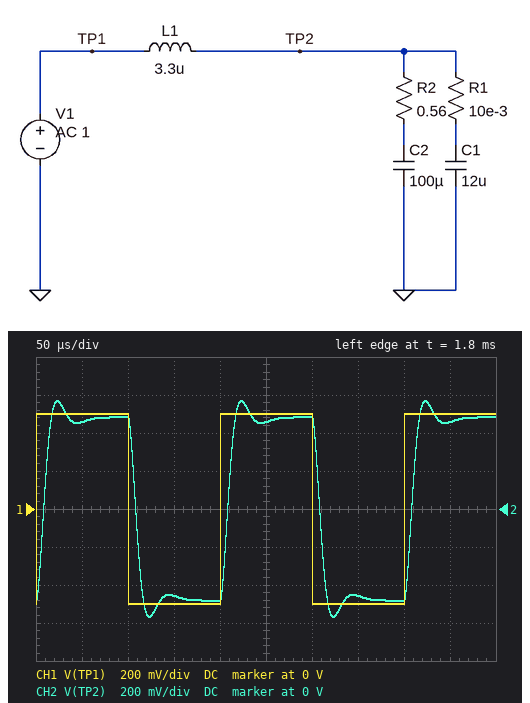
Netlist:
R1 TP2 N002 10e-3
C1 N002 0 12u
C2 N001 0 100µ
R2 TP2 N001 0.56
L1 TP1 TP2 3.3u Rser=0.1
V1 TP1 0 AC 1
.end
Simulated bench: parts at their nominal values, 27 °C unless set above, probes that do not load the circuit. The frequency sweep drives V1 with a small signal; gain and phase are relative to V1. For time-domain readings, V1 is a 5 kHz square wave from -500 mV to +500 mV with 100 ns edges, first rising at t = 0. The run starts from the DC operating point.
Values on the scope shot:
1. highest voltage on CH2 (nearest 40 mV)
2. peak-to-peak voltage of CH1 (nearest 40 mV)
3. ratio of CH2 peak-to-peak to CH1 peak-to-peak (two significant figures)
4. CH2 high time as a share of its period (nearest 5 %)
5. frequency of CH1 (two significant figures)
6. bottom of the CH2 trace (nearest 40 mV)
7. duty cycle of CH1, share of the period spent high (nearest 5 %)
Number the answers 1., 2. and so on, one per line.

1. 560 mV
2. 1.00 V
3. 1.1
4. 50 %
5. 5.0 kHz
6. -560 mV
7. 50 %
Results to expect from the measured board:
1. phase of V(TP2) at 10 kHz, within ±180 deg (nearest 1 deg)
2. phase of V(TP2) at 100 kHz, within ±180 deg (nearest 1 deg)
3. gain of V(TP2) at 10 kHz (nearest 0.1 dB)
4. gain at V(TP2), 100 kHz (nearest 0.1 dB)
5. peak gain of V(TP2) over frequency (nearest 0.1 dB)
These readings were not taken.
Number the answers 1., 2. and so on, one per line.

1. -27 deg
2. -159 deg
3. -0.2 dB
4. -23.8 dB
5. 0.1 dB
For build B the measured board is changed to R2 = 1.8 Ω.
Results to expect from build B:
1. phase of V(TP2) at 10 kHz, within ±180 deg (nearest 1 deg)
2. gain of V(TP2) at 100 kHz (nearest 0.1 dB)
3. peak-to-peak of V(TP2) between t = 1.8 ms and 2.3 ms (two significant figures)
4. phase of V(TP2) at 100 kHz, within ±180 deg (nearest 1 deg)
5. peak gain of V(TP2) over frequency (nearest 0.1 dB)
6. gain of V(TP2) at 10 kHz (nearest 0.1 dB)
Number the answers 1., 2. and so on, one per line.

1. -12 deg
2. -23.4 dB
3. 1.8 V
4. -168 deg
5. 6.1 dB
6. 0.8 dB
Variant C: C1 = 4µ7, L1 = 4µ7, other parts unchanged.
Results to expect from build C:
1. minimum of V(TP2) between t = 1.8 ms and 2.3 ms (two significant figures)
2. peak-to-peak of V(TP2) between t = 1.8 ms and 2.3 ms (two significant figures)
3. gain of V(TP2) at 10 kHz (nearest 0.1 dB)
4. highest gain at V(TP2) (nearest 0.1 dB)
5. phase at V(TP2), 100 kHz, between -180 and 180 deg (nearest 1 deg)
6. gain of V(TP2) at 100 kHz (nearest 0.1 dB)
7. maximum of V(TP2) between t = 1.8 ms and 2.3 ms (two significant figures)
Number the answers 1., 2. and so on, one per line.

1. -490 mV
2. 990 mV
3. -0.8 dB
4. 0 dB
5. -143 deg
6. -19.7 dB
7. 490 mV
